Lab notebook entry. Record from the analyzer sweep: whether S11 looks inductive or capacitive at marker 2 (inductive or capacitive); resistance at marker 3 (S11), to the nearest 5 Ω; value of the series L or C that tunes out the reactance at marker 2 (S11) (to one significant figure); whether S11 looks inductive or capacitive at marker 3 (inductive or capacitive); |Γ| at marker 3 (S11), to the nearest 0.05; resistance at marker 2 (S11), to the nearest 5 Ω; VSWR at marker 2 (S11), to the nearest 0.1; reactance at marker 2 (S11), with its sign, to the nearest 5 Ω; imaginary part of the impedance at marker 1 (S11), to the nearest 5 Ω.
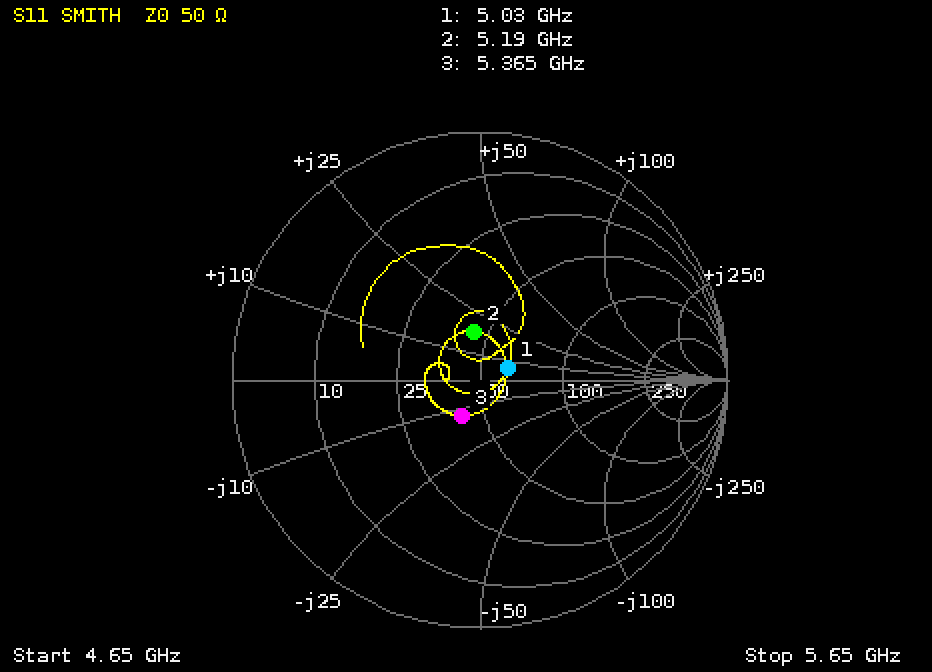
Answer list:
inductive
40 Ω
2 pF
capacitive
0.15
45 Ω
1.5
+20 Ω
+5 Ω
